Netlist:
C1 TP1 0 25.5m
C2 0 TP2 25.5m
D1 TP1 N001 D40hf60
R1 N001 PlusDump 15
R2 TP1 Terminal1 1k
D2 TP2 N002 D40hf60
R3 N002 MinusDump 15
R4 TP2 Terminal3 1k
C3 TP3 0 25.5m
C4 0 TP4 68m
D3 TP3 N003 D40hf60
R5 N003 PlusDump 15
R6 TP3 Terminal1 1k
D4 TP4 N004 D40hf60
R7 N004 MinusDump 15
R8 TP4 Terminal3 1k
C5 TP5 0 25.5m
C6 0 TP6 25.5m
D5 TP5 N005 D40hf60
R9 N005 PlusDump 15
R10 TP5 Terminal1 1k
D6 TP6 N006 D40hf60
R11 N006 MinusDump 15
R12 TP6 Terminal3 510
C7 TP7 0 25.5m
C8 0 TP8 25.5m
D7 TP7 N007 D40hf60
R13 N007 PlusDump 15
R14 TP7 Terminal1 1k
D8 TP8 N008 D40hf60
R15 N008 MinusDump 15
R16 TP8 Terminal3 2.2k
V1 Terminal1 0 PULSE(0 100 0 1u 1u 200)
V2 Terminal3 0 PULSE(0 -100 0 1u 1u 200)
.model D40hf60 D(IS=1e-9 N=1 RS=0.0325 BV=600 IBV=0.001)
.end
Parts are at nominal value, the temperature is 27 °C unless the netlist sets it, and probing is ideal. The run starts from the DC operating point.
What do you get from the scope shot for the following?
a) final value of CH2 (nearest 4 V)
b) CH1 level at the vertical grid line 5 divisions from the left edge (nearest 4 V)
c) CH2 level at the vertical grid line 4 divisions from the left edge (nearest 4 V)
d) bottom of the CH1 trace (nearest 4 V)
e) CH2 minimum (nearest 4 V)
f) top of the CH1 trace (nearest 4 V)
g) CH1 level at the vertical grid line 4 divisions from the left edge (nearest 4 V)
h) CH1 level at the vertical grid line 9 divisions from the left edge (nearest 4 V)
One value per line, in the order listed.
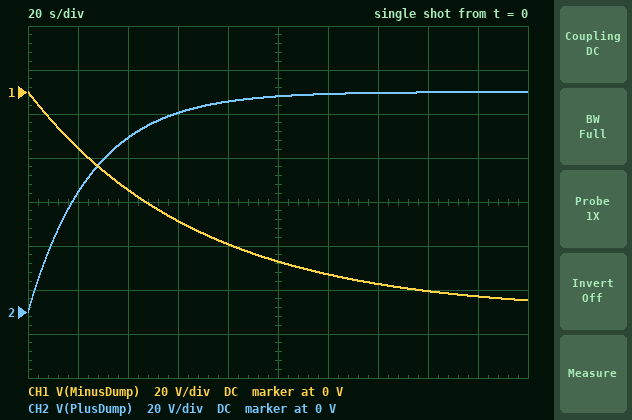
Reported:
100 V
-76 V
96 V
-96 V
0 V
0 V
-68 V
-92 V
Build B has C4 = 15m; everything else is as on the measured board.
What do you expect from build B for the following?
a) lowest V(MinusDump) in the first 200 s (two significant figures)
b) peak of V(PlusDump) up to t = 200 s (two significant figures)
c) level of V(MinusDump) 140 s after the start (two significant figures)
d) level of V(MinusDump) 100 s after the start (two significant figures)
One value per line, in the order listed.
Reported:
-97 V
100 V
-92 V
-83 V
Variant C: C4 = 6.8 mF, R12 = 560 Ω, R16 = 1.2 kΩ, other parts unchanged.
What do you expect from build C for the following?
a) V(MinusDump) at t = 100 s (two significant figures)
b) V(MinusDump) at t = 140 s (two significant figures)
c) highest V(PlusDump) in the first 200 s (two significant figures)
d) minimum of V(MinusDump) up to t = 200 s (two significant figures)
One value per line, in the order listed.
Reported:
-96 V
-99 V
100 V
-100 V
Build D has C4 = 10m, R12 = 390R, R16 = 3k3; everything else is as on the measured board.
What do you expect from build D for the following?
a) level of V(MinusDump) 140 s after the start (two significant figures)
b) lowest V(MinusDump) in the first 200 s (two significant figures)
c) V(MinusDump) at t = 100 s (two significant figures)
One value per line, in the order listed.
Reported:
-81 V
-91 V
-70 V
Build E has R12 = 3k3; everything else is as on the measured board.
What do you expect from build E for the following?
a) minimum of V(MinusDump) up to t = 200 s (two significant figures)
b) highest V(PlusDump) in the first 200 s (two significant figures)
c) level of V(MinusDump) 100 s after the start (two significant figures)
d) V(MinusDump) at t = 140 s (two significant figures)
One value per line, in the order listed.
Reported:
-91 V
100 V
-70 V
-81 V
